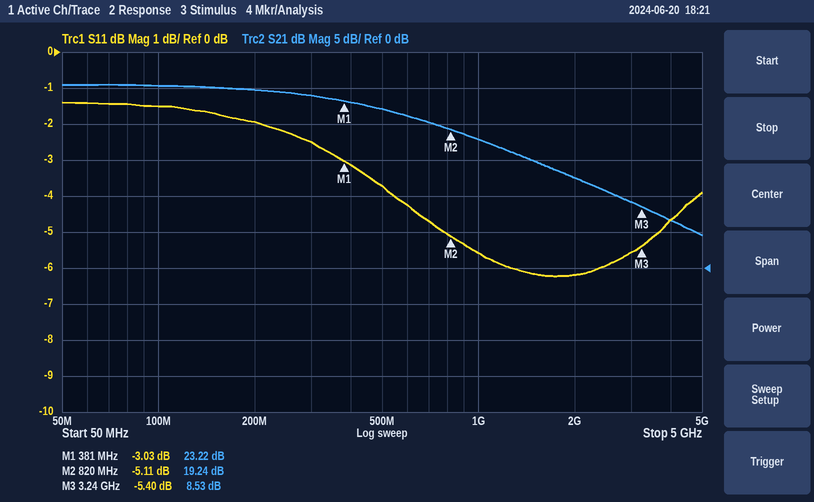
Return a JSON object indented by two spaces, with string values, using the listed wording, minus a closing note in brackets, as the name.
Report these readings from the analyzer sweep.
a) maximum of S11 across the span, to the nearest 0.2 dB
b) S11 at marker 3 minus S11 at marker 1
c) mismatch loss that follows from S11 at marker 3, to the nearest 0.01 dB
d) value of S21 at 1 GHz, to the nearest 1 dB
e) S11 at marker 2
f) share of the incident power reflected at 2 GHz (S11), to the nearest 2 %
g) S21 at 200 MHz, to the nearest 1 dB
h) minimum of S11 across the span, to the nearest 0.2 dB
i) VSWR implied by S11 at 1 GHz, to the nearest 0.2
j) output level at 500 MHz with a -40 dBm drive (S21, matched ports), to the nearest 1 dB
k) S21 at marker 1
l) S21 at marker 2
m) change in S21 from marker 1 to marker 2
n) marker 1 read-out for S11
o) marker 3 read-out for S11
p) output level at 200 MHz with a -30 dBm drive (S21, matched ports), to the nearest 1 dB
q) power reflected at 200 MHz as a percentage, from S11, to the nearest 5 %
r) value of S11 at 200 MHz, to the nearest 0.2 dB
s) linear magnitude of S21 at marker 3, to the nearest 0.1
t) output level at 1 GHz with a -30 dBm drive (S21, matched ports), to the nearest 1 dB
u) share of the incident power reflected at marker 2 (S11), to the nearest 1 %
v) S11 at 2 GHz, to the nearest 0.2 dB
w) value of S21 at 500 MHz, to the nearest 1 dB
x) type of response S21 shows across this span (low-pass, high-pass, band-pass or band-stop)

{
  "maximum of S11 across the span, to the nearest 0.2 dB": "-1.4 dB",
  "S11 at marker 3 minus S11 at marker 1": "-2.37 dB",
  "mismatch loss that follows from S11 at marker 3, to the nearest 0.01 dB": "1.48 dB",
  "value of S21 at 1 GHz, to the nearest 1 dB": "18 dB",
  "S11 at marker 2": "-5.11 dB",
  "share of the incident power reflected at 2 GHz (S11), to the nearest 2 %": "24 %",
  "S21 at 200 MHz, to the nearest 1 dB": "25 dB",
  "minimum of S11 across the span, to the nearest 0.2 dB": "-6.2 dB",
  "VSWR implied by S11 at 1 GHz, to the nearest 0.2": "3.2",
  "output level at 500 MHz with a -40 dBm drive (S21, matched ports), to the nearest 1 dB": "-18 dBm",
  "S21 at marker 1": "23.22 dB",
  "S21 at marker 2": "19.24 dB",
  "change in S21 from marker 1 to marker 2": "-3.98 dB",
  "marker 1 read-out for S11": "-3.03 dB",
  "marker 3 read-out for S11": "-5.40 dB",
  "output level at 200 MHz with a -30 dBm drive (S21, matched ports), to the nearest 1 dB": "-5 dBm",
  "power reflected at 200 MHz as a percentage, from S11, to the nearest 5 %": "65 %",
  "value of S11 at 200 MHz, to the nearest 0.2 dB": "-2.0 dB",
  "linear magnitude of S21 at marker 3, to the nearest 0.1": "2.7",
  "output level at 1 GHz with a -30 dBm drive (S21, matched ports), to the nearest 1 dB": "-12 dBm",
  "share of the incident power reflected at marker 2 (S11), to the nearest 1 %": "31 %",
  "S11 at 2 GHz, to the nearest 0.2 dB": "-6.2 dB",
  "value of S21 at 500 MHz, to the nearest 1 dB": "22 dB",
  "type of response S21 shows across this span": "low-pass"
}
